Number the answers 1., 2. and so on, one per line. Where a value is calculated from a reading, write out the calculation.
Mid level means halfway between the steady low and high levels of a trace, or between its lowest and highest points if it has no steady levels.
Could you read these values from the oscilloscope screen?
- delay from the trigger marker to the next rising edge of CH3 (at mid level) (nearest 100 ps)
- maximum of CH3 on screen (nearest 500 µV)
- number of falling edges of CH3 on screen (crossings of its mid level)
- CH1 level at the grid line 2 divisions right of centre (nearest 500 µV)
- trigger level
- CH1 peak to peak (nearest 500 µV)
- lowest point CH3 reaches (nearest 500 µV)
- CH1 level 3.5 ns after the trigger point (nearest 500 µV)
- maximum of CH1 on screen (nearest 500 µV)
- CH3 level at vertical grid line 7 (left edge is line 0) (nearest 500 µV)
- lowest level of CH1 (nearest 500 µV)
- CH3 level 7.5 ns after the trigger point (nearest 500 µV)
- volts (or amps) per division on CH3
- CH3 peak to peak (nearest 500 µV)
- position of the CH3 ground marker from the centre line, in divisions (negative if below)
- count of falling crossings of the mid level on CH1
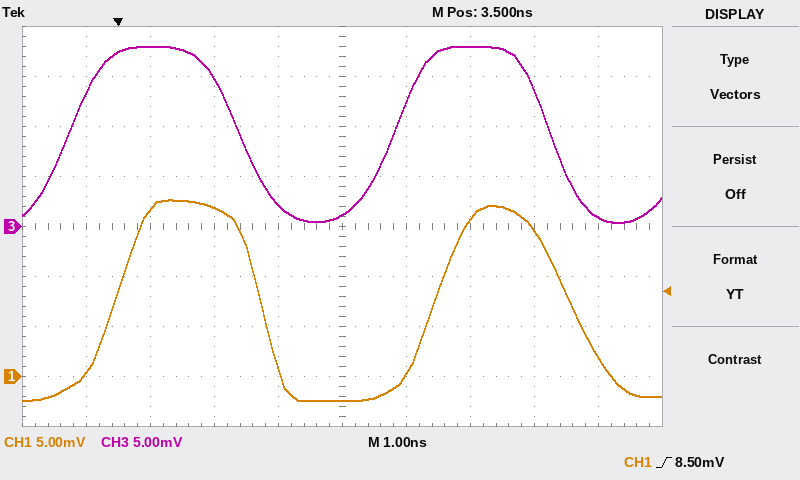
1. 4.3 ns
2. 18.0 mV
3. 2
4. 15.5 mV
5. 8.50 mV
6. 17.5 mV − (-2.5 mV) = 20.0 mV
7. 500 µV
8. -2.5 mV
9. 17.5 mV
10. 18.0 mV
11. -2.5 mV
12. 1.0 mV
13. 5 mV
14. 18.0 mV − (500 µV) = 17.5 mV
15. 0.0 div
16. 2
